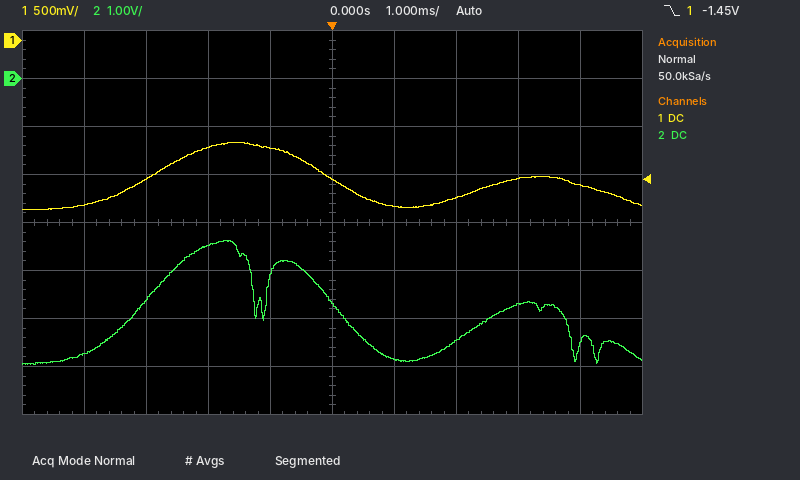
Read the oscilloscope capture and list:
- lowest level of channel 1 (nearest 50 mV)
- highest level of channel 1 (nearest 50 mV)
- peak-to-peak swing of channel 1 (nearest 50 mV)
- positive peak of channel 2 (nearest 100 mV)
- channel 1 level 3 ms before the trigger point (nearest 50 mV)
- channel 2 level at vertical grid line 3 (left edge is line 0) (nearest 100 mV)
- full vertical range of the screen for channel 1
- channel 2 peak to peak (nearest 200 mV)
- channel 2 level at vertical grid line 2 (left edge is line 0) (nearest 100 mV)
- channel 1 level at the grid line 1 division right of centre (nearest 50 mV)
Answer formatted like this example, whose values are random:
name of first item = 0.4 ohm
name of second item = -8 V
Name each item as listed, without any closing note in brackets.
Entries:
lowest level of channel 1 = -1.75 V
highest level of channel 1 = -1.05 V
peak-to-peak swing of channel 1 = 700 mV
positive peak of channel 2 = -3.4 V
channel 1 level 3 ms before the trigger point = -1.45 V
channel 2 level at vertical grid line 3 (left edge is line 0) = -3.5 V
full vertical range of the screen for channel 1 = 4 V
channel 2 peak to peak = 2.6 V
channel 2 level at vertical grid line 2 (left edge is line 0) = -4.6 V
channel 1 level at the grid line 1 division right of centre = -1.75 V
